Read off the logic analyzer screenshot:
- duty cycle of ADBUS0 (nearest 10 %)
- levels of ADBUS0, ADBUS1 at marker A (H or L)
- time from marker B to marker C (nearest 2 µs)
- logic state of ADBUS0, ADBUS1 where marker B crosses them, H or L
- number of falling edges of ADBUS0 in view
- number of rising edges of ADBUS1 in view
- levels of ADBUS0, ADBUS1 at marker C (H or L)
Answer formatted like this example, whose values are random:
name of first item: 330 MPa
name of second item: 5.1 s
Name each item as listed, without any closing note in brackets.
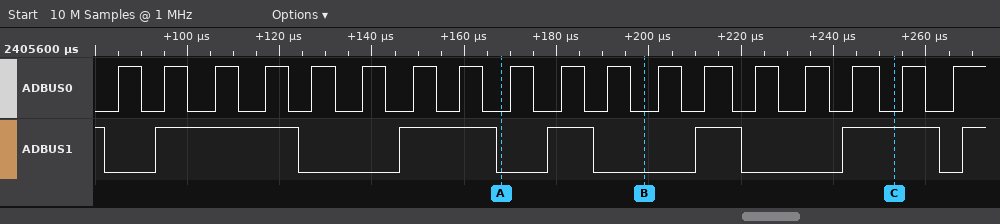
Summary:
duty cycle of ADBUS0: 50 %
levels of ADBUS0, ADBUS1 at marker A: ADBUS0=L, ADBUS1=L
time from marker B to marker C: 54 µs
logic state of ADBUS0, ADBUS1 where marker B crosses them, H or L: ADBUS0=L, ADBUS1=L
number of falling edges of ADBUS0 in view: 17
number of rising edges of ADBUS1 in view: 6
levels of ADBUS0, ADBUS1 at marker C: ADBUS0=L, ADBUS1=H
